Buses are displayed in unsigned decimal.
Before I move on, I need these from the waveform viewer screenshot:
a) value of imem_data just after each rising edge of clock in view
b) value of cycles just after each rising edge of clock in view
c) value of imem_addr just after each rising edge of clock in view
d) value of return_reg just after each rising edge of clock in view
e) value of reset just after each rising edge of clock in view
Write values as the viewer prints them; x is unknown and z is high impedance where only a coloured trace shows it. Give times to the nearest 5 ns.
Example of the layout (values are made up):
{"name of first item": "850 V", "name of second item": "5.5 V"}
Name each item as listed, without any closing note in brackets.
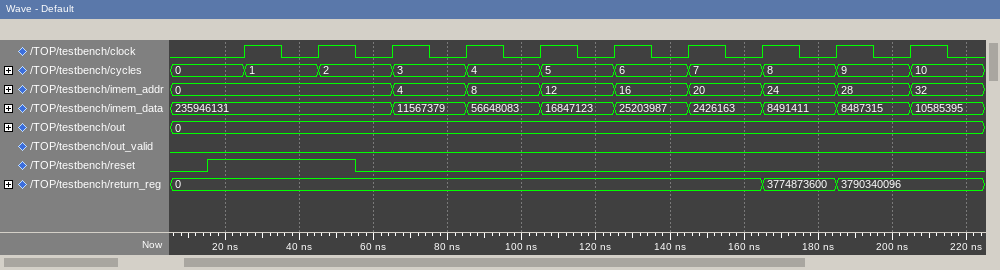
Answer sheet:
{"value of imem_data just after each rising edge of clock in view": "235946131, 235946131, 11567379, 56648083, 16847123, 25203987, 2426163, 8491411, 8487315, 10585395", "value of cycles just after each rising edge of clock in view": "1, 2, 3, 4, 5, 6, 7, 8, 9, 10", "value of imem_addr just after each rising edge of clock in view": "0, 0, 4, 8, 12, 16, 20, 24, 28, 32", "value of return_reg just after each rising edge of clock in view": "0, 0, 0, 0, 0, 0, 0, 3774873600, 3790340096, 3790340096", "value of reset just after each rising edge of clock in view": "1 1 0 0 0 0 0 0 0 0"}
